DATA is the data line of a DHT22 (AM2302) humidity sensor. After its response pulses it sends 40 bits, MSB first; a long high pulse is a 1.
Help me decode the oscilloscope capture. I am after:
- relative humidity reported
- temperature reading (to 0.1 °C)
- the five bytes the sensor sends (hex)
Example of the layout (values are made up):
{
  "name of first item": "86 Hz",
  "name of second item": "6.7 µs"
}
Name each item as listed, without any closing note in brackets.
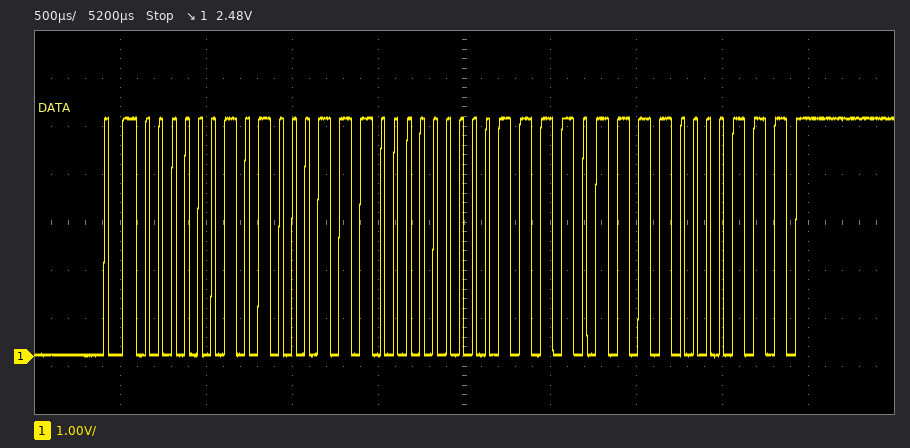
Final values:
{
  "relative humidity reported": "65.4 %",
  "temperature reading": "24.7 °C",
  "the five bytes the sensor sends": "02 8E 00 F7 87"
}
